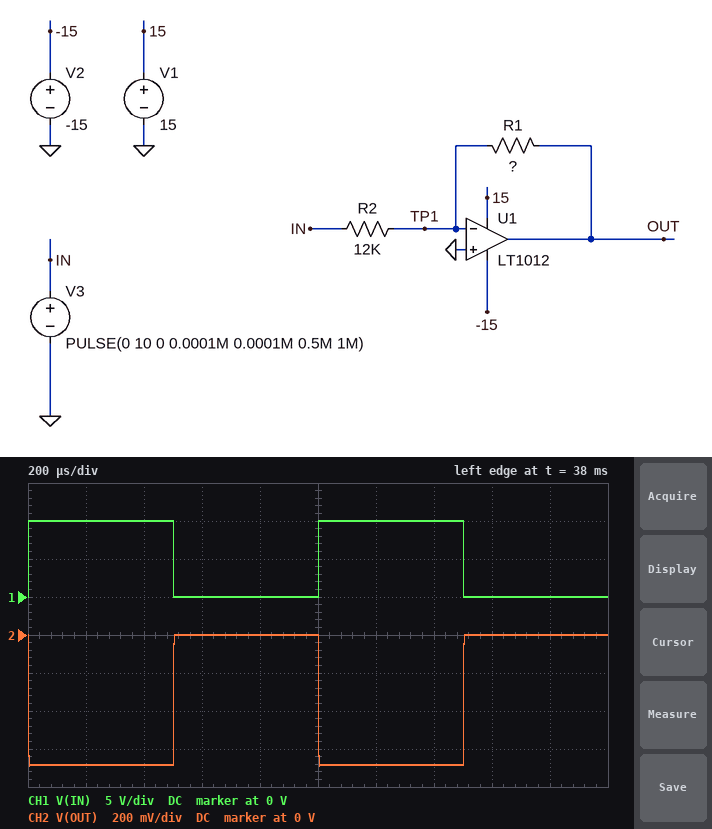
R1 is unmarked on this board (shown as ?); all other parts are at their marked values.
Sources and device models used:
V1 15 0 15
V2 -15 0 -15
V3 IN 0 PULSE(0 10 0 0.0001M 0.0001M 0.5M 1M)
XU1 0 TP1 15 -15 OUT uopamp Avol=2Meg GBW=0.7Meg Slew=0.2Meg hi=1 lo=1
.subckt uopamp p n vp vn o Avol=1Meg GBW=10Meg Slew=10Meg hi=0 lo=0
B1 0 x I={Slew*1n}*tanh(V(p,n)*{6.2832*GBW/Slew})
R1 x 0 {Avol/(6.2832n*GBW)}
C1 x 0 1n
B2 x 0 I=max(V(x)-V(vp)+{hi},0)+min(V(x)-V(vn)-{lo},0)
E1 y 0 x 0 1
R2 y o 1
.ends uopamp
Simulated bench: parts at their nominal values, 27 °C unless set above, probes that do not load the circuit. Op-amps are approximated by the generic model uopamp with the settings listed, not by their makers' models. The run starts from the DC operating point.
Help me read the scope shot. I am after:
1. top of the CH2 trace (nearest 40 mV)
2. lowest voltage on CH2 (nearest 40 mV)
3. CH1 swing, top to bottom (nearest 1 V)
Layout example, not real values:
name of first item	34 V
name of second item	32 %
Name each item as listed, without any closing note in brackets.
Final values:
top of the CH2 trace	0 V
lowest voltage on CH2	-680 mV
CH1 swing, top to bottom	10 V
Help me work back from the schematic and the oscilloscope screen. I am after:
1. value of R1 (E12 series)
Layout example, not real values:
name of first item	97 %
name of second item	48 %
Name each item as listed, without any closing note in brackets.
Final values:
value of R1	820 Ω
